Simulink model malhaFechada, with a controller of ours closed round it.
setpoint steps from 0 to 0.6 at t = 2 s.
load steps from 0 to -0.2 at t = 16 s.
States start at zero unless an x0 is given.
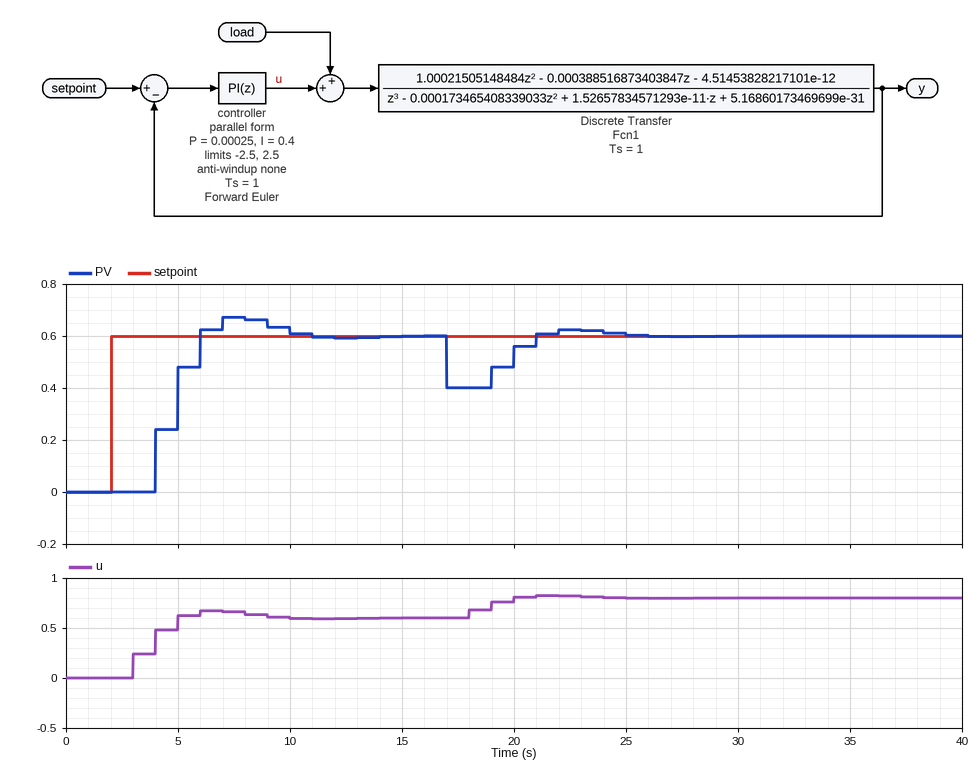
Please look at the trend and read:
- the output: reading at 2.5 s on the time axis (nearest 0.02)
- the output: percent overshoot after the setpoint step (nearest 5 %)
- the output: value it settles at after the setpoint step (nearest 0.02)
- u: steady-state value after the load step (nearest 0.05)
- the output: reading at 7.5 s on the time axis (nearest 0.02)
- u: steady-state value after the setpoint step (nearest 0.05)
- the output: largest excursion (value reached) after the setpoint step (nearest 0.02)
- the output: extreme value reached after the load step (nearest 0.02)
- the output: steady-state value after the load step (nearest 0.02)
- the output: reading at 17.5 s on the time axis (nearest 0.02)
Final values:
0.00
10 %
0.60
0.80
0.68
0.60
0.68
0.40
0.60
0.40
